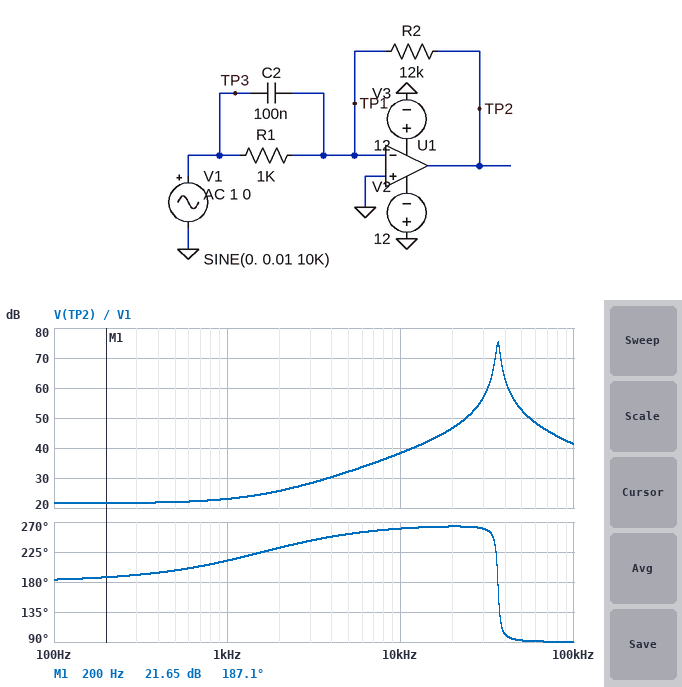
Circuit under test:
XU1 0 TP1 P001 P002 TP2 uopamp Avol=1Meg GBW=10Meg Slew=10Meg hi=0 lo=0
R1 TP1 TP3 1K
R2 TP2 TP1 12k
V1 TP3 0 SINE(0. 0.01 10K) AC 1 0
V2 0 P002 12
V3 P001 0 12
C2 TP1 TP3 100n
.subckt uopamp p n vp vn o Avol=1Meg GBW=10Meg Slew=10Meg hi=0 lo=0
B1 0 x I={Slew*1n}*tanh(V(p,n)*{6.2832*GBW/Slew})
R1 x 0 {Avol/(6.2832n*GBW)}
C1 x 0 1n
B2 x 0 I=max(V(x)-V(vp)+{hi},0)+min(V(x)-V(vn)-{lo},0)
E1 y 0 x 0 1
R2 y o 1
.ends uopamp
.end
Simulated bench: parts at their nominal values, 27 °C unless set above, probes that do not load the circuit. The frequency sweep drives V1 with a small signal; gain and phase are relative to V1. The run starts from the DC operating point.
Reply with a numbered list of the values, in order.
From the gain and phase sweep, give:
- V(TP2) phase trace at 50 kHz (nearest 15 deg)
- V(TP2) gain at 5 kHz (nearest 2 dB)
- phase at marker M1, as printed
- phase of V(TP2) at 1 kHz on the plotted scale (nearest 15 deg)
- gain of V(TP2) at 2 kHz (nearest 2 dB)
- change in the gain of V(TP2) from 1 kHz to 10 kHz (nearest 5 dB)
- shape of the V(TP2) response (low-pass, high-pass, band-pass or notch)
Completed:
1. 90 deg
2. 32 dB
3. 187.1 deg
4. 210 deg
5. 26 dB
6. 15 dB
7. band-pass
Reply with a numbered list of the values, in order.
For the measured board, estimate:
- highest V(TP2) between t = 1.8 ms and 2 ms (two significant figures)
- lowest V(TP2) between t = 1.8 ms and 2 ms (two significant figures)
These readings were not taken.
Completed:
1. 830 mV
2. -830 mV
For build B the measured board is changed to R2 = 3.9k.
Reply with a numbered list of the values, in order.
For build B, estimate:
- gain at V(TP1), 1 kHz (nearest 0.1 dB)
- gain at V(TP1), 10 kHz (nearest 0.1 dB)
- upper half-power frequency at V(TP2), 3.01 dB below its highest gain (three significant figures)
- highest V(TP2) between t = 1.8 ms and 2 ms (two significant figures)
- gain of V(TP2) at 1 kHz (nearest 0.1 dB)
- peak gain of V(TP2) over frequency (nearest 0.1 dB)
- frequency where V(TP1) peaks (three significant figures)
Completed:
1. -66.7 dB
2. -31.9 dB
3. 64.9 kHz
4. 250 mV
5. 13.3 dB
6. 73.9 dB
7. 63.9 kHz
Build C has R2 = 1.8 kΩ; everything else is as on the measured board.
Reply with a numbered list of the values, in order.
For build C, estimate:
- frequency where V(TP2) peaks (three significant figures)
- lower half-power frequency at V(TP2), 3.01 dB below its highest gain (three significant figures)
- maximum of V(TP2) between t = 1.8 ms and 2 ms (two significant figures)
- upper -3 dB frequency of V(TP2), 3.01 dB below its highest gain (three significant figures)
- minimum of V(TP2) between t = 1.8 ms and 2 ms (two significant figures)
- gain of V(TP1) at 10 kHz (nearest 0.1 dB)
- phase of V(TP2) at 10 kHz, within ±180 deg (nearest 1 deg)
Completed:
1. 94.0 kHz
2. 92.8 kHz
3. 120 mV
4. 95.3 kHz
5. -120 mV
6. -38.7 dB
7. -99 deg
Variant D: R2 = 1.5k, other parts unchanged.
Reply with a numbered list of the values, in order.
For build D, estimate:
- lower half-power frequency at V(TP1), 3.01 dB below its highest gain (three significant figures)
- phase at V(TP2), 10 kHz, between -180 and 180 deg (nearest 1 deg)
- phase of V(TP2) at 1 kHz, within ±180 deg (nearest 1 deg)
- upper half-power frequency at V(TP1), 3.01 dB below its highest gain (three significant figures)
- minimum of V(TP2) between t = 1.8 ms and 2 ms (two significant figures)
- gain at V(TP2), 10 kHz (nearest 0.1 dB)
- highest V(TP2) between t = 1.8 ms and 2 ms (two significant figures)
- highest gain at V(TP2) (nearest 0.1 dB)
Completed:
1. 102 kHz
2. -99 deg
3. -148 deg
4. 104 kHz
5. -96 mV
6. 19.7 dB
7. 96 mV
8. 71.5 dB
